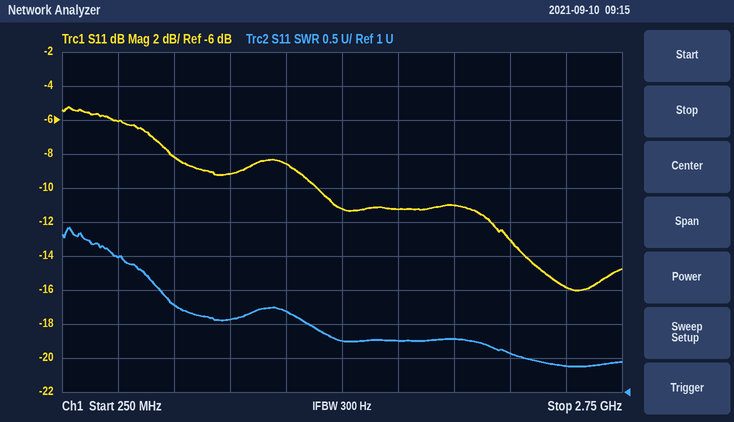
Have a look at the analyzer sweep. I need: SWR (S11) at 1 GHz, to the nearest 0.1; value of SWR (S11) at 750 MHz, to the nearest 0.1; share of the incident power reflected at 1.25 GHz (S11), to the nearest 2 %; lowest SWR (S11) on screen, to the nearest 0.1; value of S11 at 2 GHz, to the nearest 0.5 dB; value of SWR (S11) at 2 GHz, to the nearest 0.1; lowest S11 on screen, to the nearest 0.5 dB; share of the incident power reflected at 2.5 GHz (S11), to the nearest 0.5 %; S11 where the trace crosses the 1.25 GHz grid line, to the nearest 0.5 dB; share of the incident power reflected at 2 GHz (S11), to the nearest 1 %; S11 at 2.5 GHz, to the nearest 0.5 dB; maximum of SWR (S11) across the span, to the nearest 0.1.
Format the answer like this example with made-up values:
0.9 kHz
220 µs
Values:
2.1
2.3
14 %
1.4
-11.0 dB
1.8
-16.0 dB
2.5 %
-8.5 dB
8 %
-16.0 dB
3.4
